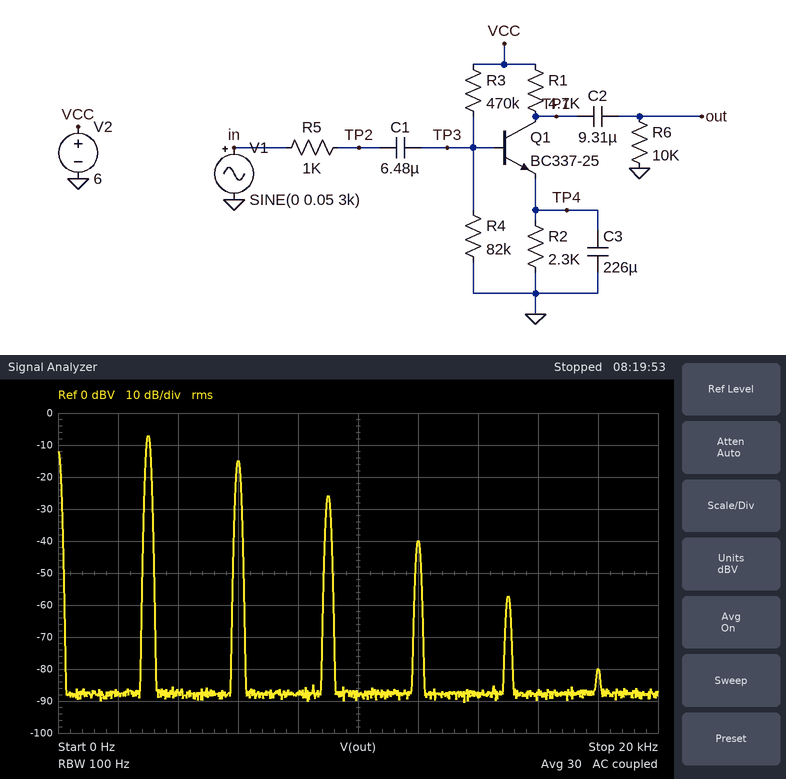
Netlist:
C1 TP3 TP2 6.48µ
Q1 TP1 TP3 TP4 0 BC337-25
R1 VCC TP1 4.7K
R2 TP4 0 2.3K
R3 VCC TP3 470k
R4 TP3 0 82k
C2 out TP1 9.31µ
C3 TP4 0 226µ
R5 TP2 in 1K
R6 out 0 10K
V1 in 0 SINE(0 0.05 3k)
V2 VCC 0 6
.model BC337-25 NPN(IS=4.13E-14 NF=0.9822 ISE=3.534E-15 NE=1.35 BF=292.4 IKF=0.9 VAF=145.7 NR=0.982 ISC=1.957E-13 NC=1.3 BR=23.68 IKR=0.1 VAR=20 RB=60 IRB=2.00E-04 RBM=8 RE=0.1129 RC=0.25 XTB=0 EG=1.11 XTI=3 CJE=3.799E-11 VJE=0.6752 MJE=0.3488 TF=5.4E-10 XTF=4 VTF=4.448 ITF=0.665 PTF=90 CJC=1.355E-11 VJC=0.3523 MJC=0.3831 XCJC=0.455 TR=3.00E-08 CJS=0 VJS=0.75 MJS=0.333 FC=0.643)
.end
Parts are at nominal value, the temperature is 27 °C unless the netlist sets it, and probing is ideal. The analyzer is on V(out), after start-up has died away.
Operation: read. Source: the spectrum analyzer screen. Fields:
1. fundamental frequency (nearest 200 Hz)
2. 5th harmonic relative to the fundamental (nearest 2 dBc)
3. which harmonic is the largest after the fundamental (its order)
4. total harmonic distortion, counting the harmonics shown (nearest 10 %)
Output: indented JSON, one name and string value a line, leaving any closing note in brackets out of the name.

{
  "fundamental frequency": "3.0 kHz",
  "5th harmonic relative to the fundamental": "-50 dBc",
  "which harmonic is the largest after the fundamental": "2",
  "total harmonic distortion, counting the harmonics shown": "40 %"
}
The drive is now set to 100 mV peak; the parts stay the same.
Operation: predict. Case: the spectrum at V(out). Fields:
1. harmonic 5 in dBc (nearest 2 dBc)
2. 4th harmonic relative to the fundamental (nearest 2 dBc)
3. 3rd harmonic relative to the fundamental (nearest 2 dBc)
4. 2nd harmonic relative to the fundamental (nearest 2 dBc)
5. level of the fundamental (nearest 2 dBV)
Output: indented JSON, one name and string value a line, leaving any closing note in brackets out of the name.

{
  "harmonic 5 in dBc": "-30 dBc",
  "4th harmonic relative to the fundamental": "-18 dBc",
  "3rd harmonic relative to the fundamental": "-10 dBc",
  "2nd harmonic relative to the fundamental": "-4 dBc",
  "level of the fundamental": "-4 dBV"
}
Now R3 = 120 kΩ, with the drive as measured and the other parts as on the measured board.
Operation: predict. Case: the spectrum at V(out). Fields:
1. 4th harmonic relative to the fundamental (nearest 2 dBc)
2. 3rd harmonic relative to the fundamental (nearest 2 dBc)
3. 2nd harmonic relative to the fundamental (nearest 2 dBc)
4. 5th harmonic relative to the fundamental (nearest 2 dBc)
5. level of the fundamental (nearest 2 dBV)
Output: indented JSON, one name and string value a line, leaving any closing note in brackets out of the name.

{
  "4th harmonic relative to the fundamental": "-30 dBc",
  "3rd harmonic relative to the fundamental": "-14 dBc",
  "2nd harmonic relative to the fundamental": "-28 dBc",
  "5th harmonic relative to the fundamental": "-24 dBc",
  "level of the fundamental": "2 dBV"
}
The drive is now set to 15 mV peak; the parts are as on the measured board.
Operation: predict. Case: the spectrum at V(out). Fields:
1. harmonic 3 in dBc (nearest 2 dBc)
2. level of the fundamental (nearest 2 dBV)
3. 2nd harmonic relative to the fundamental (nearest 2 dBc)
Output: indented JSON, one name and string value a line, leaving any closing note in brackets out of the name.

{
  "harmonic 3 in dBc": "-38 dBc",
  "level of the fundamental": "-16 dBV",
  "2nd harmonic relative to the fundamental": "-18 dBc"
}
